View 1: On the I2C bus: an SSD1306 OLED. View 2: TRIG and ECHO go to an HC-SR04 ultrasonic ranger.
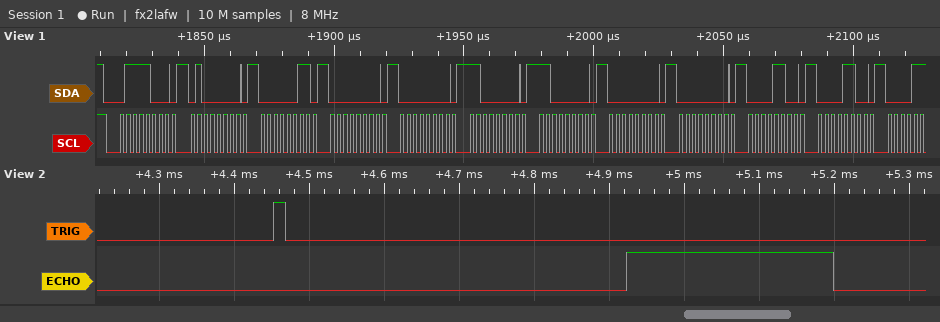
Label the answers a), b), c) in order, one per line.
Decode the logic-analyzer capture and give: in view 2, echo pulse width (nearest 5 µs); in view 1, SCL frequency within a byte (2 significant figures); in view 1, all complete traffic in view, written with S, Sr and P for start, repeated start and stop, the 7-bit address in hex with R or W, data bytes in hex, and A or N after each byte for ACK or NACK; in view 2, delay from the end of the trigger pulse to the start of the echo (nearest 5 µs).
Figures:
a) 275 µs
b) 400 kHz
c) S 3CW A 40 A 03 A 00 A 00 A C0 A C0 A 00 A 00 A 0C A 0C A
d) 455 µs
